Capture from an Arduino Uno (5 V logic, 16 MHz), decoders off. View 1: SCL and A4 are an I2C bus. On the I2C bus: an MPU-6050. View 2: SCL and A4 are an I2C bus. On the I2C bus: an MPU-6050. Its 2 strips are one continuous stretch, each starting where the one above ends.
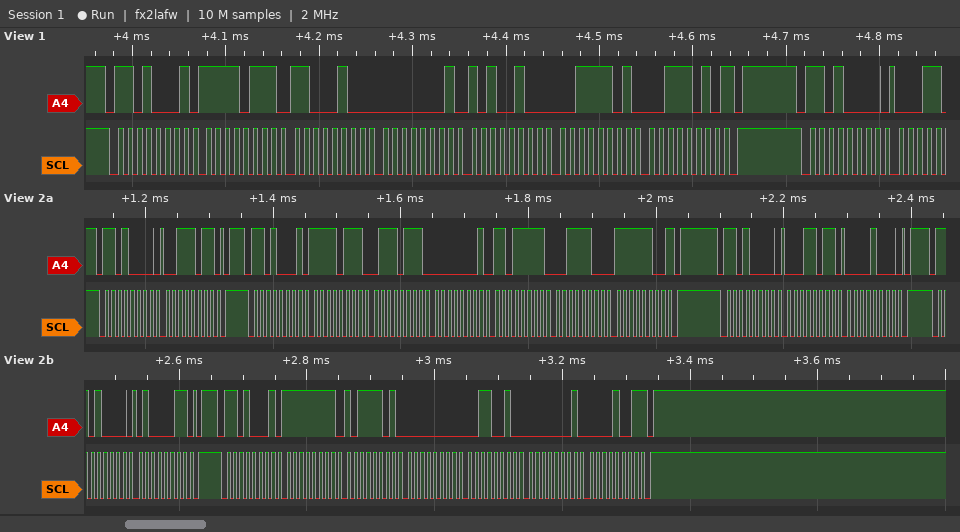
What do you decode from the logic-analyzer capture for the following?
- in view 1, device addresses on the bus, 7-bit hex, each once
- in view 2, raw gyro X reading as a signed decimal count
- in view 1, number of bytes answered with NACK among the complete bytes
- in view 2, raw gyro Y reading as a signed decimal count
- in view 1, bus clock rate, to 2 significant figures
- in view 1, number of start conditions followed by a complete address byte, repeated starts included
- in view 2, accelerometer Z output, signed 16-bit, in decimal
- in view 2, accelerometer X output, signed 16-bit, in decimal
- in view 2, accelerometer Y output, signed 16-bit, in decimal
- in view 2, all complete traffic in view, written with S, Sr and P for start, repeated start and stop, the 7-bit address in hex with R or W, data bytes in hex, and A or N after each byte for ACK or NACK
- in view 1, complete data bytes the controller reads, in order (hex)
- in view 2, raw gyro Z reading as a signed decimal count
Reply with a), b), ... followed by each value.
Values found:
a) 0x68
b) -67
c) 1
d) 50
e) 100 kHz
f) 2
g) 15612
h) -2185
i) 479
j) S 68W A 3B A P S 68R A F7 A 77 A 01 A DF A 3C A FC N P S 68W A 1B A 08 A P S 68W A 43 A P S 68R A FF A BD A 00 A 32 A 01 A 09 N P
k) F7 C4 01 A4 3D 3A
l) 265
